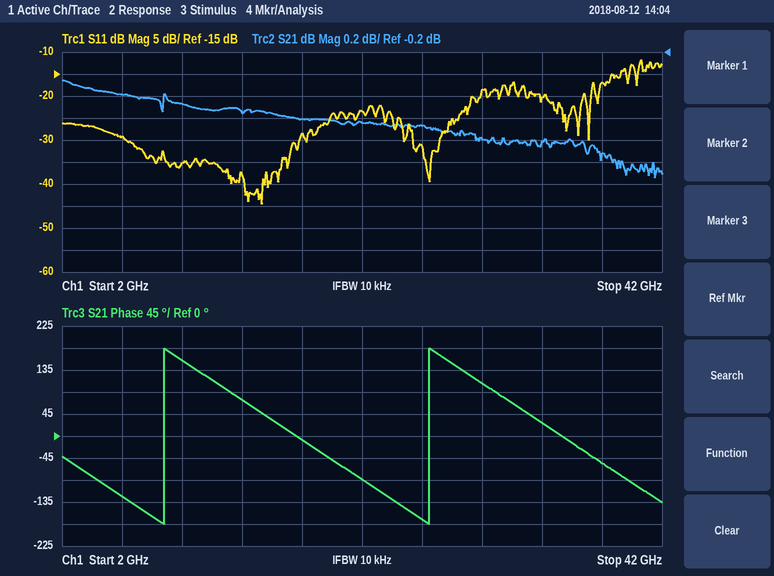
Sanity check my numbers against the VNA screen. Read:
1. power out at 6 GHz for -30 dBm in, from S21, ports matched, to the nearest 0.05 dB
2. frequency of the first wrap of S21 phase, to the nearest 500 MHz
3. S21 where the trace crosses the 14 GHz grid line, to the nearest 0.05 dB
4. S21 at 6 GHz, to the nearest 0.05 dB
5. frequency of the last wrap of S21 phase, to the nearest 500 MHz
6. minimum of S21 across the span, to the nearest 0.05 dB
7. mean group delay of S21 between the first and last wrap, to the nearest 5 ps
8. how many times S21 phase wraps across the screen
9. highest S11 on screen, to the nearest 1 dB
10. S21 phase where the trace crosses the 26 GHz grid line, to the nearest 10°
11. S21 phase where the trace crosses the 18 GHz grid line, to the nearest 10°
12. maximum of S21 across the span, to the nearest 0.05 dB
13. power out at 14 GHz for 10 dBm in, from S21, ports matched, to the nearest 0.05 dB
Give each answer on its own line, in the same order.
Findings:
-30.60 dBm
9.0 GHz
-0.75 dB
-0.60 dB
26.5 GHz
-1.35 dB
55 ps
2
-12 dB
-170°
-10°
-0.45 dB
9.25 dBm
